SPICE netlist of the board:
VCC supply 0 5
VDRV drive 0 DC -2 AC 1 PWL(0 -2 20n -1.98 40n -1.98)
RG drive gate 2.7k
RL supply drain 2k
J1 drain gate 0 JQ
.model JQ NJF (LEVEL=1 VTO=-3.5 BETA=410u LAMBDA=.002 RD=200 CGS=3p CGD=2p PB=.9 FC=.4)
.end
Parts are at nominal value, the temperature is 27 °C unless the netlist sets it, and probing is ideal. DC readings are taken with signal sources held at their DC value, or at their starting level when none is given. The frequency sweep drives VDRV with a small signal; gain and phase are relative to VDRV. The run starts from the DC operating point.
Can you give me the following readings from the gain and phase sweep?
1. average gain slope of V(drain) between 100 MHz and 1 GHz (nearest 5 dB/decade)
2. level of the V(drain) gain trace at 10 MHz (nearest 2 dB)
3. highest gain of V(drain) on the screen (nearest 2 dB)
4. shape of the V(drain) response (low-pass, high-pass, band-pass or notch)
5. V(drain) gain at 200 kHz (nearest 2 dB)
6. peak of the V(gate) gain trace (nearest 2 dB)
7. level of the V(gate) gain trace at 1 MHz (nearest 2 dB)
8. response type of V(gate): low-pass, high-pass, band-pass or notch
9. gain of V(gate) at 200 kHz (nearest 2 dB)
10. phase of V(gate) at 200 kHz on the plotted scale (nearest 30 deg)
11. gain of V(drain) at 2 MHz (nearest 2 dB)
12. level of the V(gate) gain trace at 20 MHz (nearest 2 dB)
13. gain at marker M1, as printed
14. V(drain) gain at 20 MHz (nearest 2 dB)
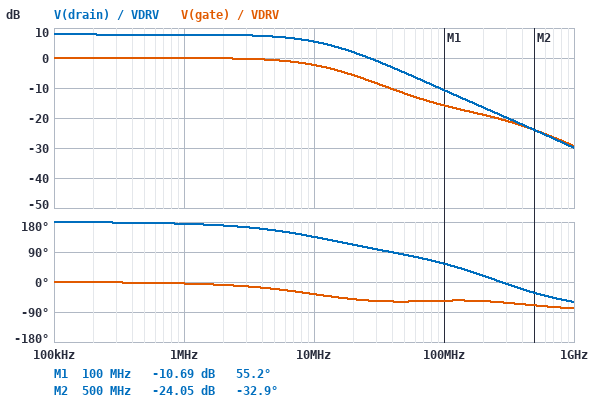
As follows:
-20 dB/decade
6 dB
8 dB
low-pass
8 dB
0 dB
0 dB
low-pass
0 dB
0 deg
8 dB
-6 dB
-10.69 dB
2 dB
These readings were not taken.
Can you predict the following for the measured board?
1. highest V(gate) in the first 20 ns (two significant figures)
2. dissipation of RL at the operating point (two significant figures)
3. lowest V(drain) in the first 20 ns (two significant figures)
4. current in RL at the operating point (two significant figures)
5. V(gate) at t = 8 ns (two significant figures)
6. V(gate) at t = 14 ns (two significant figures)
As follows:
-2.0 V
1.7 mW
3.1 V
930 µA
-2.0 V
-2.0 V
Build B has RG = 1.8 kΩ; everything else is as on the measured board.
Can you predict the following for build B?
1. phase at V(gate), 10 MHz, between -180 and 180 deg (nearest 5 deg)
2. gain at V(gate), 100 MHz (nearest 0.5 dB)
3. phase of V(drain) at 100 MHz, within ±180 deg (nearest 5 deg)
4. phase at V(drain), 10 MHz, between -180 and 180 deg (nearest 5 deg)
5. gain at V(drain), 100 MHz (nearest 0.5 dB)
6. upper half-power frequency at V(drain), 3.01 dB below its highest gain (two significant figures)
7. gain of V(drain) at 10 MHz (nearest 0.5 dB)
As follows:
-25 deg
-12.5 dB
60 deg
145 deg
-7.5 dB
17 MHz
6.5 dB
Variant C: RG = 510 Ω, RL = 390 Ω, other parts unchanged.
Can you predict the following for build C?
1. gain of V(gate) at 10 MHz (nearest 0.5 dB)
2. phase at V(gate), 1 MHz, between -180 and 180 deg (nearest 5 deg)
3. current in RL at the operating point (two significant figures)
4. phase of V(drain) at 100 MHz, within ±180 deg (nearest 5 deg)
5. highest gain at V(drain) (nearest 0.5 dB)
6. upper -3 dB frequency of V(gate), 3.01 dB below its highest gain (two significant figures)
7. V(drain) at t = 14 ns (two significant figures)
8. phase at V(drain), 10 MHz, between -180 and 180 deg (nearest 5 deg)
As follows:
0 dB
0 deg
930 µA
105 deg
-6.5 dB
100 MHz
4.6 V
170 deg
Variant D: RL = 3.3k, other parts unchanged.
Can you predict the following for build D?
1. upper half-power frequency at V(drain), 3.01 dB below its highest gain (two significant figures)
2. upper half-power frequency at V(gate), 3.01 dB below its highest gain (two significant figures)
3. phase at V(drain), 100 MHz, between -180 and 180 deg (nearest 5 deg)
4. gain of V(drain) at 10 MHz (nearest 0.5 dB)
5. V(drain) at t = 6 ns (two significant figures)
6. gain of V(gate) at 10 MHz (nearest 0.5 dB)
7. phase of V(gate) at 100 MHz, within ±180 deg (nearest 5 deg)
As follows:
8.2 MHz
8.4 MHz
45 deg
8.0 dB
1.9 V
-4.0 dB
-45 deg
